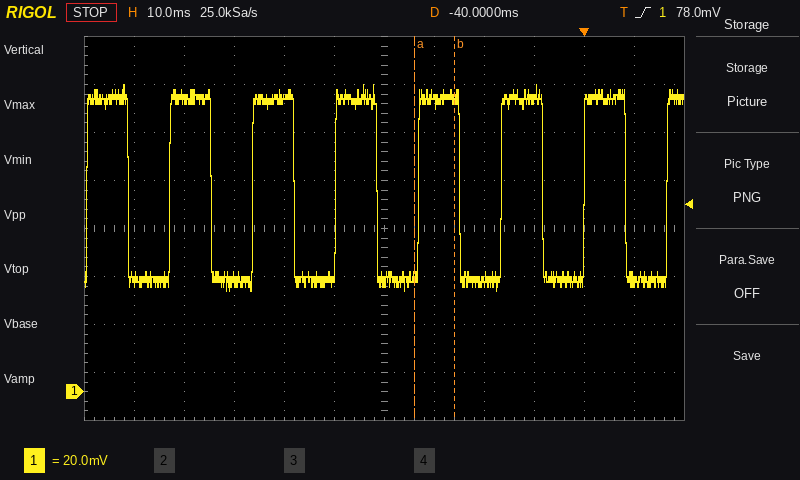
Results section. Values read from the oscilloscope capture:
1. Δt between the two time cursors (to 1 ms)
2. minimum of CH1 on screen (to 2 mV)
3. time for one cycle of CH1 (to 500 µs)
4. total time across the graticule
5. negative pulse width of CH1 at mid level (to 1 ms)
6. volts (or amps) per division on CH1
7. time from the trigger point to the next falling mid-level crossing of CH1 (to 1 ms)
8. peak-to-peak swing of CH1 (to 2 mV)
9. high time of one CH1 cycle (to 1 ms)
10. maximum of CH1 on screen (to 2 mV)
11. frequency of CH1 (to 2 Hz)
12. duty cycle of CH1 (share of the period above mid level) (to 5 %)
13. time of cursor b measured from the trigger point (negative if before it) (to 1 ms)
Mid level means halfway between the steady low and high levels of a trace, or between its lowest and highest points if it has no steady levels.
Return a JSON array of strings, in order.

["8 ms", "42 mV", "16.5 ms", "120 ms", "8 ms", "20 mV", "8 ms", "86 mV", "8 ms", "128 mV", "60 Hz", "50 %", "-26 ms"]
